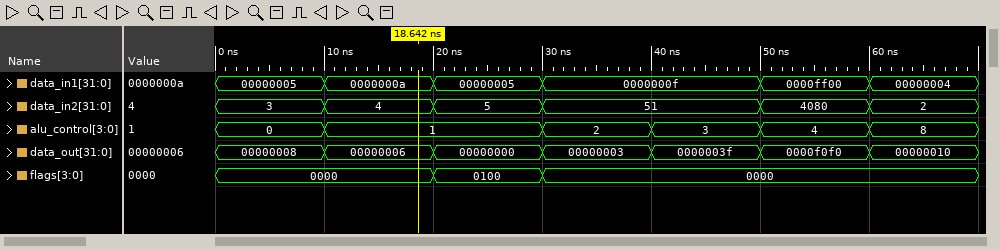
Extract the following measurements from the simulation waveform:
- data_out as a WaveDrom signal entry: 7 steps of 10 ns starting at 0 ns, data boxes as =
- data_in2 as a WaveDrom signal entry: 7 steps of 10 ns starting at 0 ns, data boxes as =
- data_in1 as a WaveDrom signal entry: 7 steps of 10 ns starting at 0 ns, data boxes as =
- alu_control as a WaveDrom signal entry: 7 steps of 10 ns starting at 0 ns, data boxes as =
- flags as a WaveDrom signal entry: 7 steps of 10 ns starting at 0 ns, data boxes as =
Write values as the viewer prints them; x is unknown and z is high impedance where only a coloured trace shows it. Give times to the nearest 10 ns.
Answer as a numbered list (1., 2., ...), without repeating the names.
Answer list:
1. {name: 'data_out', wave: '=======', data: '00000008 00000006 00000000 00000003 0000003f 0000f0f0 00000010'}
2. {name: 'data_in2', wave: '====.==', data: '3 4 5 51 4080 2'}
3. {name: 'data_in1', wave: '====.==', data: '00000005 0000000a 00000005 0000000f 0000ff00 00000004'}
4. {name: 'alu_control', wave: '==.====', data: '0 1 2 3 4 8'}
5. {name: 'flags', wave: '=.==...', data: '0000 0100 0000'}
